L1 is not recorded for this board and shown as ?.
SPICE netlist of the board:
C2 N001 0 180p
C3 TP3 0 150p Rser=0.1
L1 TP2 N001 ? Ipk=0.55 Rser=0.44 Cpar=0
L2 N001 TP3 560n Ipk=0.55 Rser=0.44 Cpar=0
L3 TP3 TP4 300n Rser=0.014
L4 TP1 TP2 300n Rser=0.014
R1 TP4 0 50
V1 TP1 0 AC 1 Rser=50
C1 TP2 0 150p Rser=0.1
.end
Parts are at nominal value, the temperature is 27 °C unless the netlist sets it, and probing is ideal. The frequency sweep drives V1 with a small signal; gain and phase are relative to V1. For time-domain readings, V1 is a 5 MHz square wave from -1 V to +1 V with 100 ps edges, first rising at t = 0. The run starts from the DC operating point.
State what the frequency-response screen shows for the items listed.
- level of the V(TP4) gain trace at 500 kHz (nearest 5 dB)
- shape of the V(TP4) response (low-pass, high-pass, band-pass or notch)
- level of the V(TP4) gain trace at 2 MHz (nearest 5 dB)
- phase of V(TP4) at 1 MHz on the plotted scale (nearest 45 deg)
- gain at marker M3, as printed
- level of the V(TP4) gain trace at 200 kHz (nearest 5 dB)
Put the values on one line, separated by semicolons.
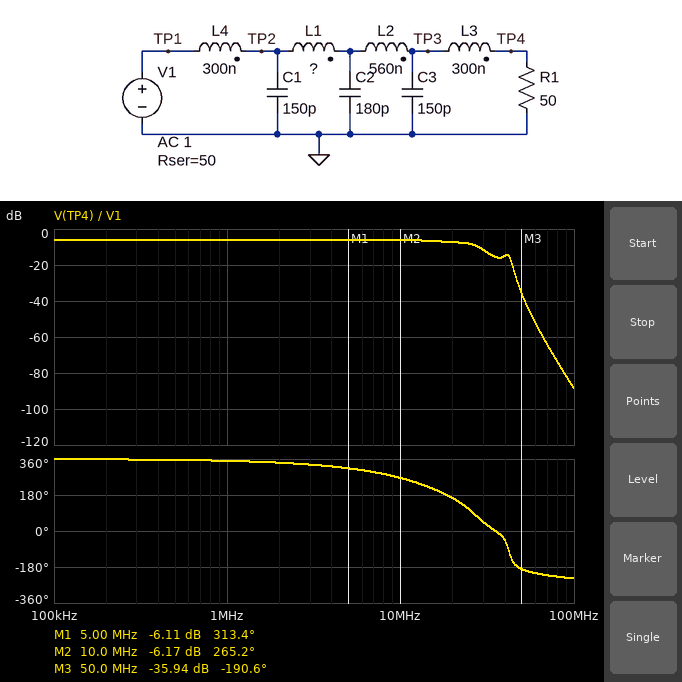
-5 dB; low-pass; -5 dB; 360 deg; -35.94 dB; -5 dB
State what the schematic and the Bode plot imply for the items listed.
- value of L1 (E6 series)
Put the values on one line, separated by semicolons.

220 nH
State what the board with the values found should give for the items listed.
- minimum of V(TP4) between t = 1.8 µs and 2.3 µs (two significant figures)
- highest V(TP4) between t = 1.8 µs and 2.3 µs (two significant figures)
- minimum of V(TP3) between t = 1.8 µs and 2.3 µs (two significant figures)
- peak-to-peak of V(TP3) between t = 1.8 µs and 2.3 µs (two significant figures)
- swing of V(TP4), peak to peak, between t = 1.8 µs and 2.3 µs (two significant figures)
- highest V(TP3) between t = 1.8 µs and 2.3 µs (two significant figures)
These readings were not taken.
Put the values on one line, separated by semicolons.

-590 mV; 590 mV; -700 mV; 1.4 V; 1.2 V; 700 mV
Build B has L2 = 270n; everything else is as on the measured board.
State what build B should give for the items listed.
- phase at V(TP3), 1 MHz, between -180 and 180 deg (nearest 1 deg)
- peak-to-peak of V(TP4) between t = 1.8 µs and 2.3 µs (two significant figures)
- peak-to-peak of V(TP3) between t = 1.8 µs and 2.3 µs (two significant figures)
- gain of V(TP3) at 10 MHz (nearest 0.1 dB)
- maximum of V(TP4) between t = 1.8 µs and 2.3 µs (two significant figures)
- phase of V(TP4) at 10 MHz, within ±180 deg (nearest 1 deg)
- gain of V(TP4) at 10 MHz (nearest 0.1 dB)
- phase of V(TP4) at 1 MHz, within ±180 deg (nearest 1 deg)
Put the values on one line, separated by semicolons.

-6 deg; 1.2 V; 1.6 V; -5.7 dB; 610 mV; -84 deg; -6.3 dB; -8 deg
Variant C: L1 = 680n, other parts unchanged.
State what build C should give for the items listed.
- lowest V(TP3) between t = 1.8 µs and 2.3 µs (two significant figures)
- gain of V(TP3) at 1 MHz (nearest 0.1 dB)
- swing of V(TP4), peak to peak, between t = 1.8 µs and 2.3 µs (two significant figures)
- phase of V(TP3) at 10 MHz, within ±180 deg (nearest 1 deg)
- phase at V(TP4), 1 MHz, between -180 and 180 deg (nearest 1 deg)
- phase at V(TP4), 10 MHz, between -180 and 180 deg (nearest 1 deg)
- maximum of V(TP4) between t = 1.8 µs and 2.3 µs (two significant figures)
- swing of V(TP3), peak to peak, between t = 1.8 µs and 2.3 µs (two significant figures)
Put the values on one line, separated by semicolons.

-750 mV; -6.1 dB; 1.3 V; -88 deg; -11 deg; -109 deg; 650 mV; 1.5 V
